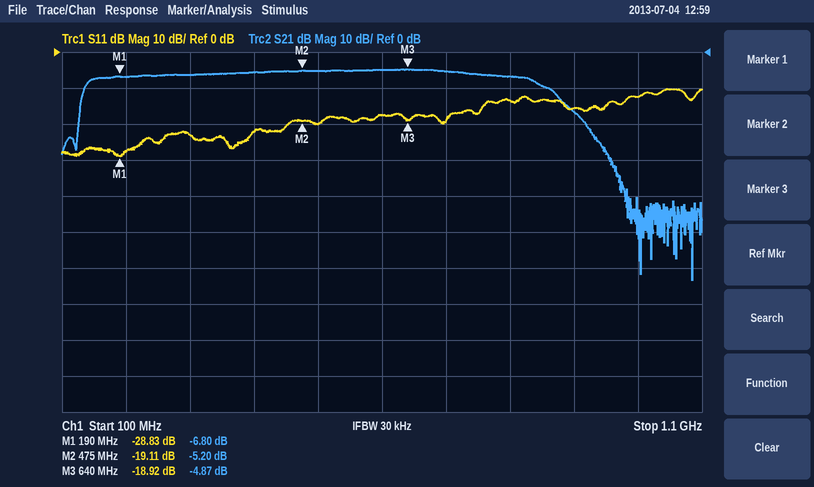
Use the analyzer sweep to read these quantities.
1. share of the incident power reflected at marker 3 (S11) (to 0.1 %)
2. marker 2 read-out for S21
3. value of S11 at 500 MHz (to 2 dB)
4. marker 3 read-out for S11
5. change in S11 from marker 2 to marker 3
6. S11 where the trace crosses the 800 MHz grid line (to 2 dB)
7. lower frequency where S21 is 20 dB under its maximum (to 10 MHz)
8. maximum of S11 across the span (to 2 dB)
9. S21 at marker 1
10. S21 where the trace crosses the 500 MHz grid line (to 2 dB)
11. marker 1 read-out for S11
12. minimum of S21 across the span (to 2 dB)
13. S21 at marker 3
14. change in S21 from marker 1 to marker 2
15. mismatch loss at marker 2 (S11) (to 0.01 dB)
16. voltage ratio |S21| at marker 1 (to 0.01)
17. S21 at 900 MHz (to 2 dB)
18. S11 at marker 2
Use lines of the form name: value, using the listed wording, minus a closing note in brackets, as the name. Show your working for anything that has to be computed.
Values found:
share of the incident power reflected at marker 3 (S11): 10^(-18.92/10) ≈ 1.3 %
marker 2 read-out for S21: -5.20 dB
value of S11 at 500 MHz: -20 dB
marker 3 read-out for S11: -18.92 dB
change in S11 from marker 2 to marker 3: -18.92 − (-19.11) = 0.19 dB
S11 where the trace crosses the 800 MHz grid line: -14 dB
lower frequency where S21 is 20 dB under its maximum: 120 MHz
maximum of S11 across the span: -10 dB
S21 at marker 1: -6.80 dB
S21 where the trace crosses the 500 MHz grid line: -6 dB
marker 1 read-out for S11: -28.83 dB
minimum of S21 across the span: -64 dB
S21 at marker 3: -4.87 dB
change in S21 from marker 1 to marker 2: -5.2 − (-6.8) = 1.60 dB
mismatch loss at marker 2 (S11): −10 log10(1 − 10^(-19.11/10)) ≈ 0.05 dB
voltage ratio |S21| at marker 1: 10^(-6.8/20) ≈ 0.46
S21 at 900 MHz: -16 dB
S11 at marker 2: -19.11 dB
